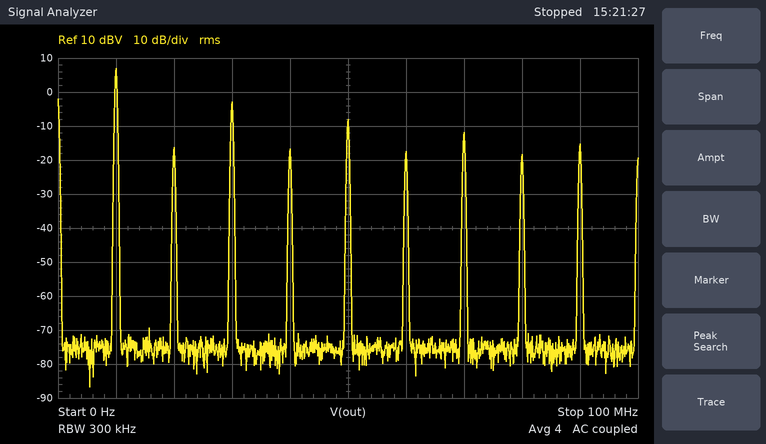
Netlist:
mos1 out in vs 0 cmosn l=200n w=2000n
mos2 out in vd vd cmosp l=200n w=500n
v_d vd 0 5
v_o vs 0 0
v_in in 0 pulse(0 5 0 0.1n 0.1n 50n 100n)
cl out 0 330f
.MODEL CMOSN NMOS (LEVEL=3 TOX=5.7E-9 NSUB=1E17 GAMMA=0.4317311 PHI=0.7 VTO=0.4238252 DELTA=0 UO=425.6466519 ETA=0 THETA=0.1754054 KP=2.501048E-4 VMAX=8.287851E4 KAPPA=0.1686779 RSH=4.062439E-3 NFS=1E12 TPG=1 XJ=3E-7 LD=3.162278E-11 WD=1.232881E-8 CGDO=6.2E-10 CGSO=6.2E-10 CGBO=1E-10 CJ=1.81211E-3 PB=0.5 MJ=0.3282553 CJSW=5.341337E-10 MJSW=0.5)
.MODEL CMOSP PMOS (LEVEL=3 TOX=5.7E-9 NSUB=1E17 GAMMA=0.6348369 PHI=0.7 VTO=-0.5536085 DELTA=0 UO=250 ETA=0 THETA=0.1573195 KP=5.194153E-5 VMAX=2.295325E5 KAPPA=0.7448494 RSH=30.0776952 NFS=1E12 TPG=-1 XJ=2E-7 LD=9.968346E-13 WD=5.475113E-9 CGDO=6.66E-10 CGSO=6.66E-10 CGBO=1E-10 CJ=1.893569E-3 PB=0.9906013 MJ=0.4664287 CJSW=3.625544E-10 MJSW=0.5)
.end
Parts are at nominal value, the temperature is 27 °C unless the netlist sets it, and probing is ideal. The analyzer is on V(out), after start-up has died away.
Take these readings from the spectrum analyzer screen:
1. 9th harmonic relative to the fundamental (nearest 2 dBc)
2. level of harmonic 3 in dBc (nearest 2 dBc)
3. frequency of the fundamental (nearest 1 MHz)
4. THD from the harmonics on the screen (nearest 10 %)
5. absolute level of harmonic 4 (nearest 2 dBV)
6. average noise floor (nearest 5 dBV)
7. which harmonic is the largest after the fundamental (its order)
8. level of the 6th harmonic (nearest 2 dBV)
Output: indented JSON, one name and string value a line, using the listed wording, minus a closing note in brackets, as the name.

{
  "9th harmonic relative to the fundamental": "-22 dBc",
  "level of harmonic 3 in dBc": "-10 dBc",
  "frequency of the fundamental": "10 MHz",
  "THD from the harmonics on the screen": "40 %",
  "absolute level of harmonic 4": "-16 dBV",
  "average noise floor": "-75 dBV",
  "which harmonic is the largest after the fundamental": "3",
  "level of the 6th harmonic": "-18 dBV"
}
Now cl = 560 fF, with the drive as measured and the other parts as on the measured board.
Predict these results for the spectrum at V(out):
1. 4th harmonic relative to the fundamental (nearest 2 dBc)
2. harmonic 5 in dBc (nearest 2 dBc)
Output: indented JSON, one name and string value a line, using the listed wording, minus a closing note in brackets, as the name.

{
  "4th harmonic relative to the fundamental": "-20 dBc",
  "harmonic 5 in dBc": "-16 dBc"
}
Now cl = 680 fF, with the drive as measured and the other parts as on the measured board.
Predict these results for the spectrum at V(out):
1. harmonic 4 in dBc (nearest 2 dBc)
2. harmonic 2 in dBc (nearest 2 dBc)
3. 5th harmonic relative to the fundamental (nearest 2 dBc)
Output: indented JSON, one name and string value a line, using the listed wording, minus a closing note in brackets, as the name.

{
  "harmonic 4 in dBc": "-20 dBc",
  "harmonic 2 in dBc": "-18 dBc",
  "5th harmonic relative to the fundamental": "-18 dBc"
}
